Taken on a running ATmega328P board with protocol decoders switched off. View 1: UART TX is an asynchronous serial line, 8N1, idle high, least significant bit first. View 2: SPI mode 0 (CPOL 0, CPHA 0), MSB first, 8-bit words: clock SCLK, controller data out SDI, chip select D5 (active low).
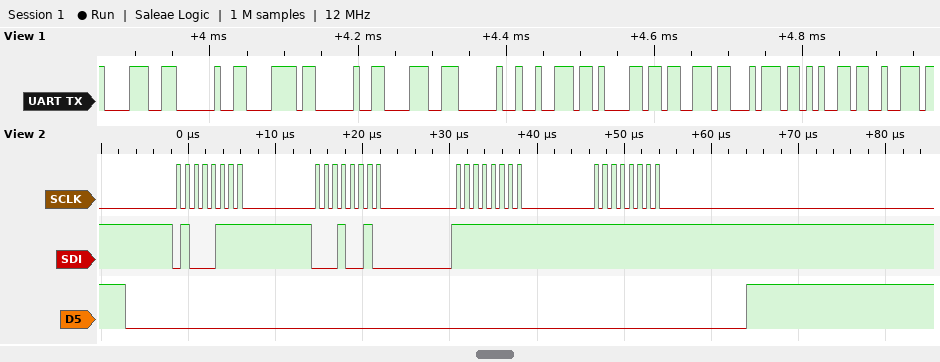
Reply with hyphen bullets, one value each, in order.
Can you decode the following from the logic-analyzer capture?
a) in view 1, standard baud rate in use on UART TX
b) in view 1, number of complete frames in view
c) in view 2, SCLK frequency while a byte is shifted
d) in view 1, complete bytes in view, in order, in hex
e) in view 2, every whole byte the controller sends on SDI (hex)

- 115200 baud
- 12
- 1 MHz
- 38 20 78 20 38 20 72 61 73 74 65 72
- 0x47 0x12 0xFF 0xFF
